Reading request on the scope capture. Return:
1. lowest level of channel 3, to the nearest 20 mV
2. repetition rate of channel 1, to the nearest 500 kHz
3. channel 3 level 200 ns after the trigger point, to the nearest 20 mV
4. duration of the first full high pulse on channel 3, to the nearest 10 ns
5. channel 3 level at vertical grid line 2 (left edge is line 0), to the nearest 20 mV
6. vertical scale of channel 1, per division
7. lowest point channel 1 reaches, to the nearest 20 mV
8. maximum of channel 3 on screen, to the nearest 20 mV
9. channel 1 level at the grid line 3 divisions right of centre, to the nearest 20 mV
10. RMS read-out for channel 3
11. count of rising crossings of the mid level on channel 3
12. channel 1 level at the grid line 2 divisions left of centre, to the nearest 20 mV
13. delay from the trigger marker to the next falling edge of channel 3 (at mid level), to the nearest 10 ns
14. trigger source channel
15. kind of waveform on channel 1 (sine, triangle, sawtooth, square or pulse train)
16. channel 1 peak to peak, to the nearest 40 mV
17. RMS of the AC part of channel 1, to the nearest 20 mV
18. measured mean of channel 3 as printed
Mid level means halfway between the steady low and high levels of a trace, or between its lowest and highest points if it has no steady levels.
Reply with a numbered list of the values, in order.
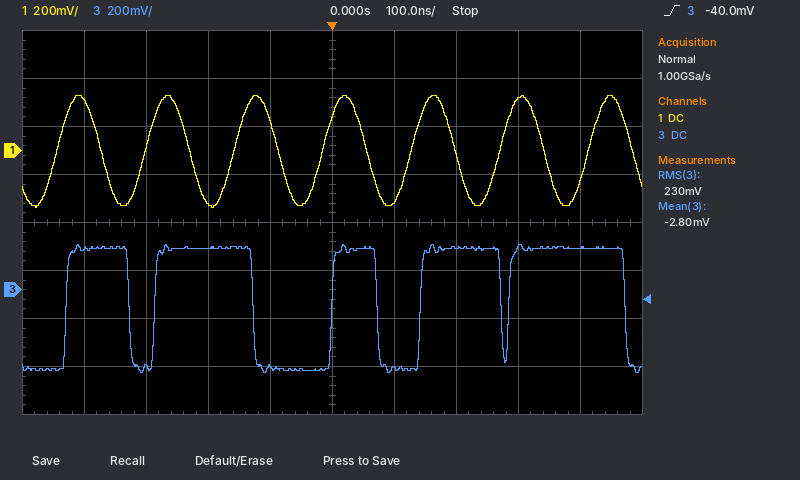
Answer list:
1. -340 mV
2. 7.0 MHz
3. 180 mV
4. 100 ns
5. -320 mV
6. 200 mV
7. -240 mV
8. 180 mV
9. 220 mV
10. 230 mV
11. 5
12. -220 mV
13. 70 ns
14. channel 3
15. sine
16. 480 mV
17. 160 mV
18. -2.80 mV
